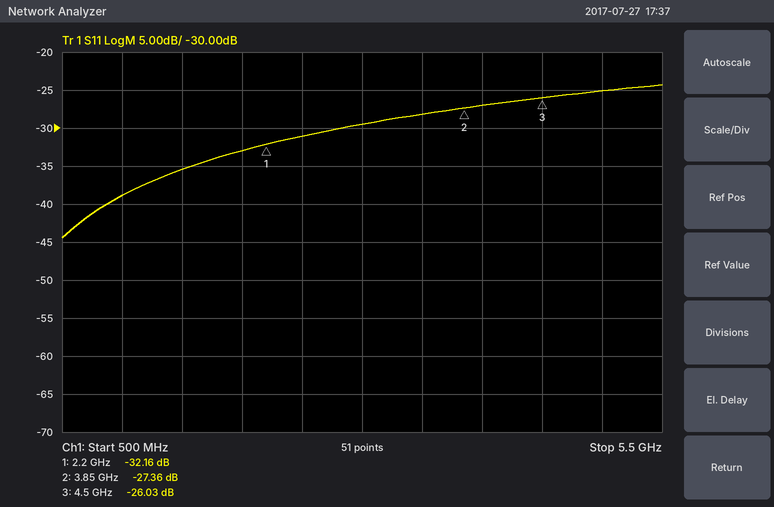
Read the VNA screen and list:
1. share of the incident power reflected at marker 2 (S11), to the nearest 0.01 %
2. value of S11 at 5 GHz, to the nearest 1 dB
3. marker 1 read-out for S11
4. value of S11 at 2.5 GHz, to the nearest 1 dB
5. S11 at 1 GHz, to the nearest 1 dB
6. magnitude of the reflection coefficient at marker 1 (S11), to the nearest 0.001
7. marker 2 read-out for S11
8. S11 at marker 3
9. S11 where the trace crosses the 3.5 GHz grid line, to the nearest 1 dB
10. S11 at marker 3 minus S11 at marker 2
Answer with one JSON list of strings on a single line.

["0.18 %", "-25 dB", "-32.16 dB", "-31 dB", "-39 dB", "0.025", "-27.36 dB", "-26.03 dB", "-28 dB", "1.33 dB"]
